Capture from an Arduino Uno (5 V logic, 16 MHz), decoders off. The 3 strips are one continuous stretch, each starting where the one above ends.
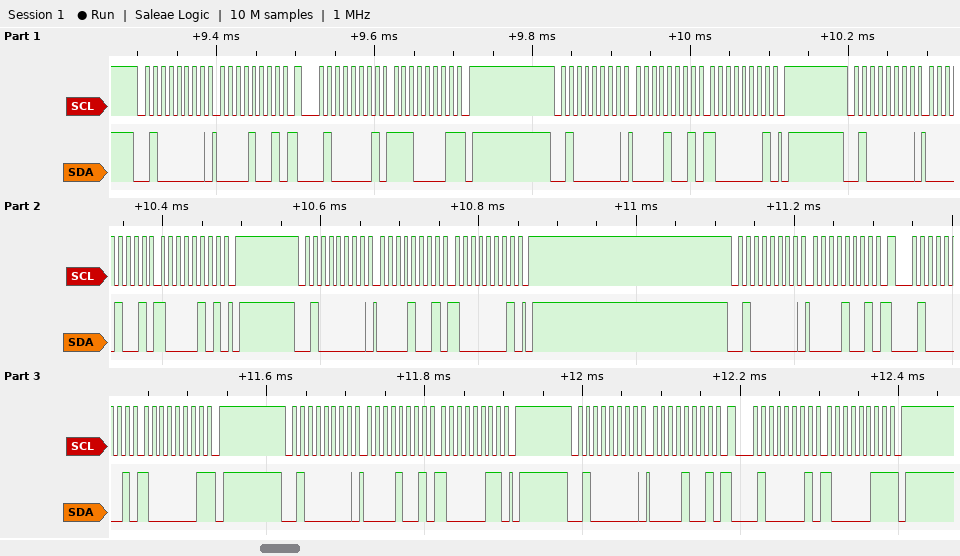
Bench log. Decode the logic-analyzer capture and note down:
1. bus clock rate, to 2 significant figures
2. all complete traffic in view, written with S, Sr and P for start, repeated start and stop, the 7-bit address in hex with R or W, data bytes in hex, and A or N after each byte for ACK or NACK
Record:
100 kHz
S 20W A 09 A Sr 20R A E1 N P S 20W A 09 A 81 A P S 20W A 09 A 85 A P S 20W A 09 A 81 A P S 20W A 09 A Sr 20R A 81 N P S 20W A 09 A 83 A P S 20W A 09 A Sr 20R A 83 N P
